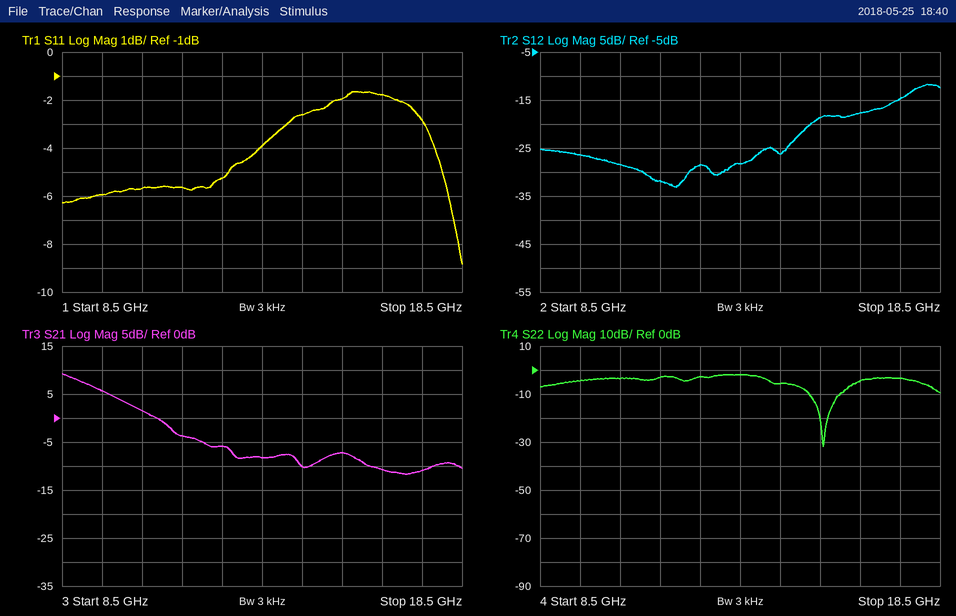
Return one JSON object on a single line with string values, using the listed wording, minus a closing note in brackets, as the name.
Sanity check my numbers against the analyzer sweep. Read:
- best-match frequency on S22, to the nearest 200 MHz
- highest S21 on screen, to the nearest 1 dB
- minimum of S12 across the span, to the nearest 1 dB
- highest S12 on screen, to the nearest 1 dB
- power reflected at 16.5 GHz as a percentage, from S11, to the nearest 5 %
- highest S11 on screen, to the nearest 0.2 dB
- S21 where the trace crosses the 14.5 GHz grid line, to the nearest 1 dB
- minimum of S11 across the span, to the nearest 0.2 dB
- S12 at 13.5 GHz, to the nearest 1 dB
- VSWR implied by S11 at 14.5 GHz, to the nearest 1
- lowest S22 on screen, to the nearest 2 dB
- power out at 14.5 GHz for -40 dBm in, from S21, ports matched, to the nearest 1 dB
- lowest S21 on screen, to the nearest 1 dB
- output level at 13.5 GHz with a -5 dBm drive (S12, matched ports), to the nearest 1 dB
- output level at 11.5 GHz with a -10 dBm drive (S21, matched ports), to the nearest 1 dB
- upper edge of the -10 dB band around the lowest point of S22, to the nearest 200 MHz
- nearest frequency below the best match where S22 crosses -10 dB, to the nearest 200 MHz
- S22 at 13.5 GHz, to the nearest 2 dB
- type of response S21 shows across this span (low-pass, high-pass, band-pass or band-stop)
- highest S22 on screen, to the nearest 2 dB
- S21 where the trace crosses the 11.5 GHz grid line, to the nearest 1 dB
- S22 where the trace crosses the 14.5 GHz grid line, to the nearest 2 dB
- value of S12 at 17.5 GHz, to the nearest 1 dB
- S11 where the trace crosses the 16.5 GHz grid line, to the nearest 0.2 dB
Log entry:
{"best-match frequency on S22, to the nearest 200 MHz": "15.6 GHz", "highest S21 on screen, to the nearest 1 dB": "9 dB", "minimum of S12 across the span, to the nearest 1 dB": "-33 dB", "highest S12 on screen, to the nearest 1 dB": "-12 dB", "power reflected at 16.5 GHz as a percentage, from S11, to the nearest 5 %": "65 %", "highest S11 on screen, to the nearest 0.2 dB": "-1.6 dB", "S21 where the trace crosses the 14.5 GHz grid line, to the nearest 1 dB": "-10 dB", "minimum of S11 across the span, to the nearest 0.2 dB": "-8.8 dB", "S12 at 13.5 GHz, to the nearest 1 dB": "-28 dB", "VSWR implied by S11 at 14.5 GHz, to the nearest 1": "7", "lowest S22 on screen, to the nearest 2 dB": "-32 dB", "power out at 14.5 GHz for -40 dBm in, from S21, ports matched, to the nearest 1 dB": "-50 dBm", "lowest S21 on screen, to the nearest 1 dB": "-12 dB", "output level at 13.5 GHz with a -5 dBm drive (S12, matched ports), to the nearest 1 dB": "-33 dBm", "output level at 11.5 GHz with a -10 dBm drive (S21, matched ports), to the nearest 1 dB": "-14 dBm", "upper edge of the -10 dB band around the lowest point of S22, to the nearest 200 MHz": "16.0 GHz", "nearest frequency below the best match where S22 crosses -10 dB, to the nearest 200 MHz": "15.2 GHz", "S22 at 13.5 GHz, to the nearest 2 dB": "-2 dB", "type of response S21 shows across this span": "low-pass", "highest S22 on screen, to the nearest 2 dB": "-2 dB", "S21 where the trace crosses the 11.5 GHz grid line, to the nearest 1 dB": "-4 dB", "S22 where the trace crosses the 14.5 GHz grid line, to the nearest 2 dB": "-6 dB", "value of S12 at 17.5 GHz, to the nearest 1 dB": "-15 dB", "S11 where the trace crosses the 16.5 GHz grid line, to the nearest 0.2 dB": "-1.8 dB"}
